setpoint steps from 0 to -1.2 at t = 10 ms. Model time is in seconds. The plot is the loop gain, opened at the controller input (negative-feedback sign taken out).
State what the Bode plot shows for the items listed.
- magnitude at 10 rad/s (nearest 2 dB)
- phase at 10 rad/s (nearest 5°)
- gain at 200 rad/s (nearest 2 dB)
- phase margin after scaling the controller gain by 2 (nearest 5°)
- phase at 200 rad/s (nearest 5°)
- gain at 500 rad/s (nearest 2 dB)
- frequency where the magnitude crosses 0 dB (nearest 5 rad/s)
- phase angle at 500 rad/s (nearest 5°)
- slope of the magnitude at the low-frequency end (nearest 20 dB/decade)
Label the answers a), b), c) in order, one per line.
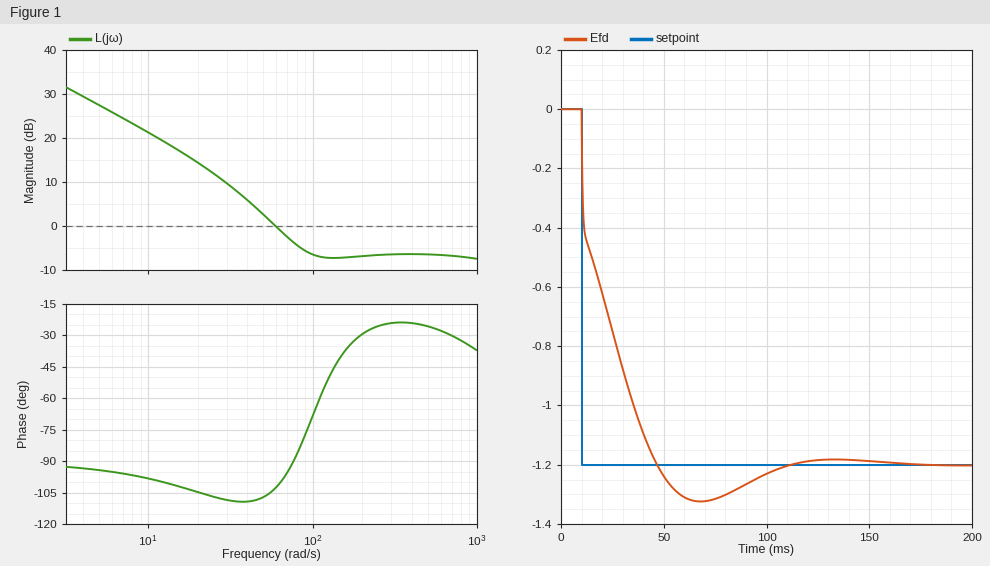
a) 22 dB
b) -100°
c) -6 dB
d) 105°
e) -30°
f) -6 dB
g) 60 rad/s
h) -25°
i) -20 dB/decade
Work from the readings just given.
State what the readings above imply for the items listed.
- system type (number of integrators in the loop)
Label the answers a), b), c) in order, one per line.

a) 1
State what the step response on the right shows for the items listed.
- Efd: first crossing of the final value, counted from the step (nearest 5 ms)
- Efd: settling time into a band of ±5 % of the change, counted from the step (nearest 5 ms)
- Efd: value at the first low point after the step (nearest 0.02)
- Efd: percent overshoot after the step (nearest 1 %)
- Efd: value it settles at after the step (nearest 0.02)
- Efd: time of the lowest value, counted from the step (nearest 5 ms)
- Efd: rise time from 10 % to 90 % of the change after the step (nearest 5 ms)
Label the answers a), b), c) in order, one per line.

a) 35 ms
b) 80 ms
c) -1.32
d) 10 %
e) -1.20
f) 60 ms
g) 30 ms
